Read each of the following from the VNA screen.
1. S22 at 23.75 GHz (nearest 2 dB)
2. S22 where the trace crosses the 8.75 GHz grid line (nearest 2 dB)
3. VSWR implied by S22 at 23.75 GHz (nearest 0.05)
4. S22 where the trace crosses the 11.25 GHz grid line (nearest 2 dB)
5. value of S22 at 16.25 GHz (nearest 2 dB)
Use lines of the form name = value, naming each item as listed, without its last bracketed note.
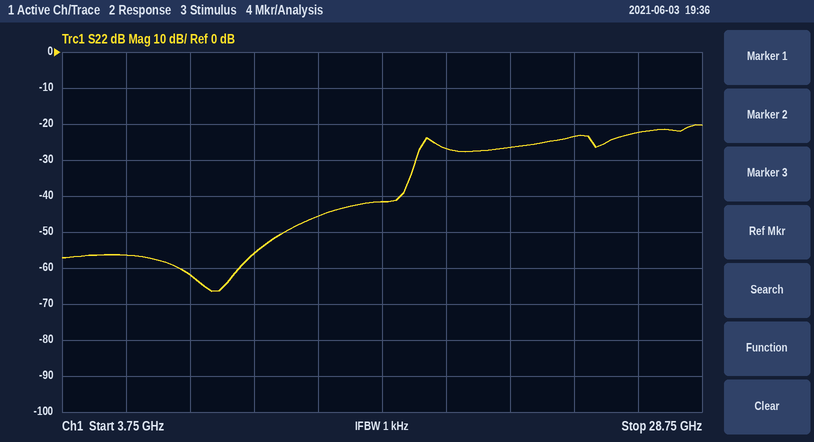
S22 at 23.75 GHz = -24 dB
S22 where the trace crosses the 8.75 GHz grid line = -62 dB
VSWR implied by S22 at 23.75 GHz = 1.15
S22 where the trace crosses the 11.25 GHz grid line = -56 dB
value of S22 at 16.25 GHz = -42 dB
